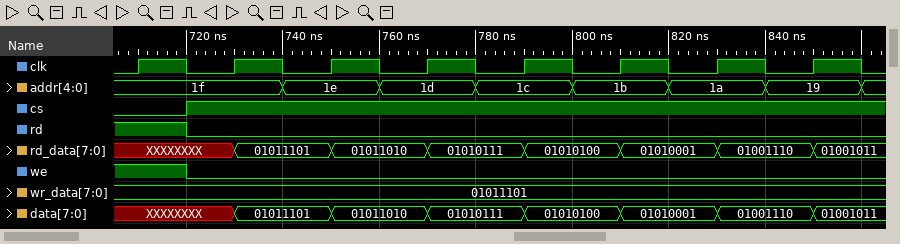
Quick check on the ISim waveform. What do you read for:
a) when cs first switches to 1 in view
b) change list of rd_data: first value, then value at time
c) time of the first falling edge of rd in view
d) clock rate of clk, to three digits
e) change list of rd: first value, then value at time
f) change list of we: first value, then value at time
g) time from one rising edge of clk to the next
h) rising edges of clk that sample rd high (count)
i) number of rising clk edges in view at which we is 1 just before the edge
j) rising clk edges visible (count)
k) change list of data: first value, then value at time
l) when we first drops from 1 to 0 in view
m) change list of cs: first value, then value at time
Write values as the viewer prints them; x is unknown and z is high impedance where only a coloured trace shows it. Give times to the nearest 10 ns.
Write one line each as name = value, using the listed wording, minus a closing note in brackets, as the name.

when cs first switches to 1 in view = 720 ns
change list of rd_data: first value, then value at time = XXXXXXXX, 01011101 at 730 ns, 01011010 at 750 ns, 01010111 at 770 ns, 01010100 at 790 ns, 01010001 at 810 ns, 01001110 at 830 ns, 01001011 at 850 ns
time of the first falling edge of rd in view = 720 ns
clock rate of clk, to three digits = 50.0 MHz
change list of rd: first value, then value at time = 1, 0 at 720 ns
change list of we: first value, then value at time = 1, 0 at 720 ns
time from one rising edge of clk to the next = 20 ns
rising edges of clk that sample rd high = 1
number of rising clk edges in view at which we is 1 just before the edge = 1
rising clk edges visible = 8
change list of data: first value, then value at time = XXXXXXXX, 01011101 at 730 ns, 01011010 at 750 ns, 01010111 at 770 ns, 01010100 at 790 ns, 01010001 at 810 ns, 01001110 at 830 ns, 01001011 at 850 ns
when we first drops from 1 to 0 in view = 720 ns
change list of cs: first value, then value at time = 0, 1 at 720 ns
